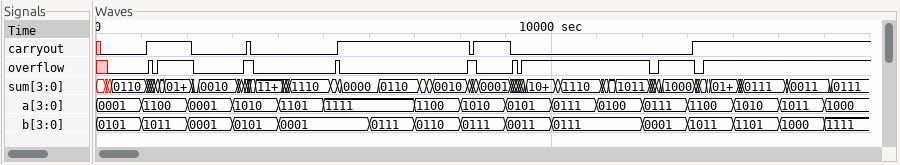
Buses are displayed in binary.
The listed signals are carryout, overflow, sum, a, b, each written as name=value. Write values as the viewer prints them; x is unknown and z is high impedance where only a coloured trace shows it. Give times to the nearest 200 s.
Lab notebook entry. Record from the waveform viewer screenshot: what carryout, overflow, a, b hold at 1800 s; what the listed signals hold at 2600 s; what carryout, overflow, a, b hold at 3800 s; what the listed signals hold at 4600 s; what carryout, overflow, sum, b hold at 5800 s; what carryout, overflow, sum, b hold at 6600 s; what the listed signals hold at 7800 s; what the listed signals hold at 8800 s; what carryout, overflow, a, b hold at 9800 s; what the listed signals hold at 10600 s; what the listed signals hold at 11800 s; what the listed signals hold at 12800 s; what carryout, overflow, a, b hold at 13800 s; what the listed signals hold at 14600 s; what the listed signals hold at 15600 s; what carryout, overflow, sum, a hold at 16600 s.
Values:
carryout=1, overflow=1, a=1100, b=1011
carryout=0, overflow=0, sum=0010, a=0001, b=0001
carryout=0, overflow=0, a=1010, b=0101
carryout=0, overflow=0, sum=1110, a=1101, b=0001
carryout=1, overflow=0, sum=0000, b=0001
carryout=1, overflow=0, sum=0110, b=0111
carryout=1, overflow=0, sum=0010, a=1100, b=0110
carryout=1, overflow=0, sum=0001, a=1010, b=0111
carryout=0, overflow=1, a=0101, b=0011
carryout=0, overflow=1, sum=1110, a=0111, b=0111
carryout=0, overflow=1, sum=1011, a=0100, b=0111
carryout=0, overflow=1, sum=1000, a=0111, b=0001
carryout=1, overflow=1, a=1100, b=1011
carryout=1, overflow=1, sum=0111, a=1010, b=1101
carryout=1, overflow=1, sum=0011, a=1011, b=1000
carryout=1, overflow=1, sum=0111, a=1000
